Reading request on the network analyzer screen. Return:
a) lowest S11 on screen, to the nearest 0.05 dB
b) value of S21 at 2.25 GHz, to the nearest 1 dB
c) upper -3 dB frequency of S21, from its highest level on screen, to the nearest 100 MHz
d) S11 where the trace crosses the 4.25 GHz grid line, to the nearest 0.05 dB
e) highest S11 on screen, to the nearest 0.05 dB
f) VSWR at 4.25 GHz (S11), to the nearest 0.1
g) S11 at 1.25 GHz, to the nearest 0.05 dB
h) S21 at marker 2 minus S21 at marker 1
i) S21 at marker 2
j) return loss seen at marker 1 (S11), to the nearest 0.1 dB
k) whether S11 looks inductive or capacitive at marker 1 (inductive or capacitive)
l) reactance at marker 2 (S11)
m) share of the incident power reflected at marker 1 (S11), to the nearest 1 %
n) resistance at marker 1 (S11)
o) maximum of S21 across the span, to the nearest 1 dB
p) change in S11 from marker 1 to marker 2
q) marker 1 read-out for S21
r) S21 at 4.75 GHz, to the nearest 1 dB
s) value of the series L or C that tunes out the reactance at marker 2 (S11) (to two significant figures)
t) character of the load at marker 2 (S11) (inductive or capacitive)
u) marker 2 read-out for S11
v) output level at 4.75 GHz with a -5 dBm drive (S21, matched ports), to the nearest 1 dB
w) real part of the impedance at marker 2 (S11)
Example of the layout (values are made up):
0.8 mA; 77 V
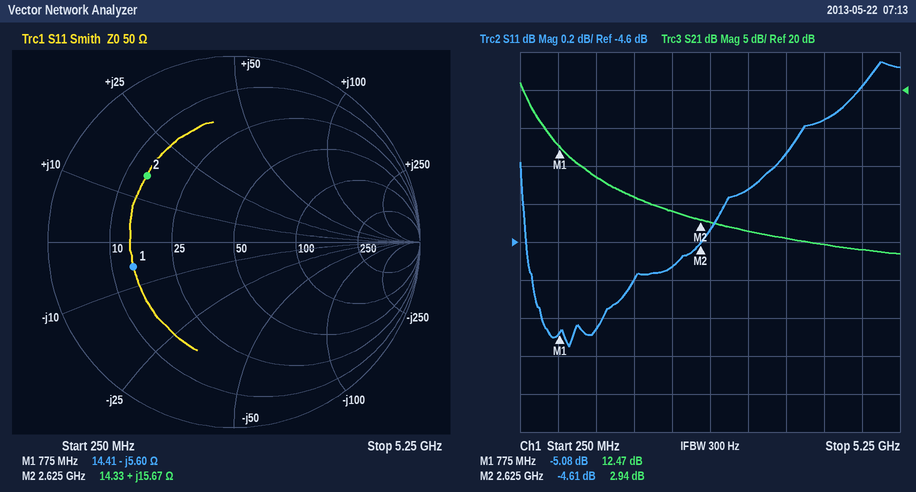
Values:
-5.15 dB; 4 dB; 400 MHz; -3.95 dB; -3.65 dB; 4.5; -5.05 dB; -9.53 dB; 2.94 dB; 5.1 dB; capacitive; +15.67 Ω; 31 %; 14.41 Ω; 21 dB; 0.47 dB; 12.47 dB; -1 dB; 3.9 pF; inductive; -4.61 dB; -6 dBm; 14.33 Ω
